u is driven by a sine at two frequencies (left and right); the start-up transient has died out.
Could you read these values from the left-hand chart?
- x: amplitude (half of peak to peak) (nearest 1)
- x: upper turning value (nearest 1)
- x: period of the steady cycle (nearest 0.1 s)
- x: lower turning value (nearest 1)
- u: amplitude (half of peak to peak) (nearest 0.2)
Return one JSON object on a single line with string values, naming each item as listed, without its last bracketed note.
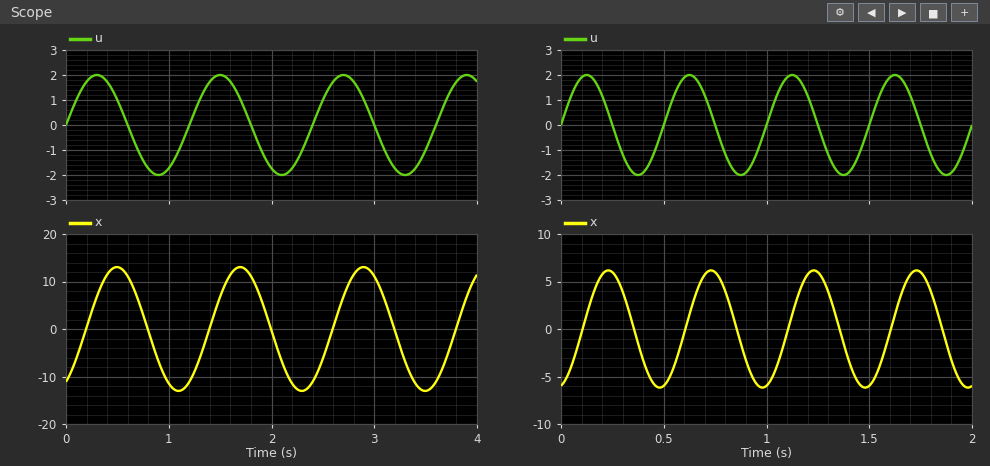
{"x: amplitude (half of peak to peak)": "13", "x: upper turning value": "13", "x: period of the steady cycle": "1.2 s", "x: lower turning value": "-13", "u: amplitude (half of peak to peak)": "2.0"}
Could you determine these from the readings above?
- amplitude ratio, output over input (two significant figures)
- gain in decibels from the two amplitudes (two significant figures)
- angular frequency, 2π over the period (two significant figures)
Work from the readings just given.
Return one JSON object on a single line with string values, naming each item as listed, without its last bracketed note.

{"amplitude ratio, output over input": "6.5", "gain in decibels from the two amplitudes": "16 dB", "angular frequency, 2π over the period": "5.2 rad/s"}
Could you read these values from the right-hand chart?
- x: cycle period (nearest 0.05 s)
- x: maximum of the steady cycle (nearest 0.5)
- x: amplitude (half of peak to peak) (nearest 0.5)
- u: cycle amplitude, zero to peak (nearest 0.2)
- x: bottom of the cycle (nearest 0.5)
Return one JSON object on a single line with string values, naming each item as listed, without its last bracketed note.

{"x: cycle period": "0.50 s", "x: maximum of the steady cycle": "6.0", "x: amplitude (half of peak to peak)": "6.0", "u: cycle amplitude, zero to peak": "2.0", "x: bottom of the cycle": "-6.0"}
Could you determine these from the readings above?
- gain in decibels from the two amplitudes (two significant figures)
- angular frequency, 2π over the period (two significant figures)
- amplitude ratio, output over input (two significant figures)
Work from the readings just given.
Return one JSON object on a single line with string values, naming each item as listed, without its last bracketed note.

{"gain in decibels from the two amplitudes": "9.5 dB", "angular frequency, 2π over the period": "13 rad/s", "amplitude ratio, output over input": "3.0"}
